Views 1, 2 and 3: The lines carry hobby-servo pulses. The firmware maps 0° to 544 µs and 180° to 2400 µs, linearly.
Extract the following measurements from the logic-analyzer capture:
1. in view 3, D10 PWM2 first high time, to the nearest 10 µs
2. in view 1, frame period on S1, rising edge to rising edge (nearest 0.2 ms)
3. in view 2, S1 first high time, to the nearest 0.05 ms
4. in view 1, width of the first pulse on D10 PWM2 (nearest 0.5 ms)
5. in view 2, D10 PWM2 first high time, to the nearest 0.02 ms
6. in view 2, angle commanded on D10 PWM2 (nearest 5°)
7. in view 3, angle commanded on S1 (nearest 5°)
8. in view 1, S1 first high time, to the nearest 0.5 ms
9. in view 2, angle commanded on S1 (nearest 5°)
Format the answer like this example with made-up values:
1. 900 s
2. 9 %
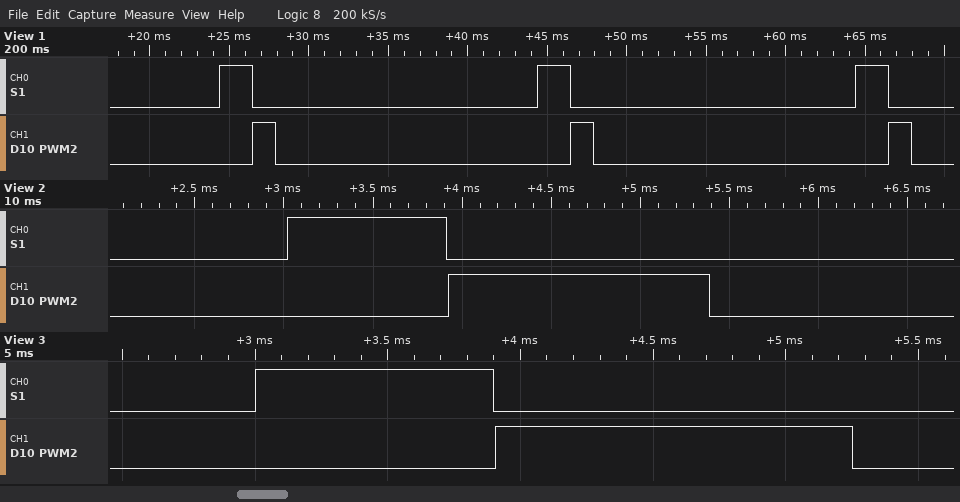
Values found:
1. 1350 µs
2. 20.0 ms
3. 0.90 ms
4. 1.5 ms
5. 1.46 ms
6. 90°
7. 35°
8. 2.0 ms
9. 35°
